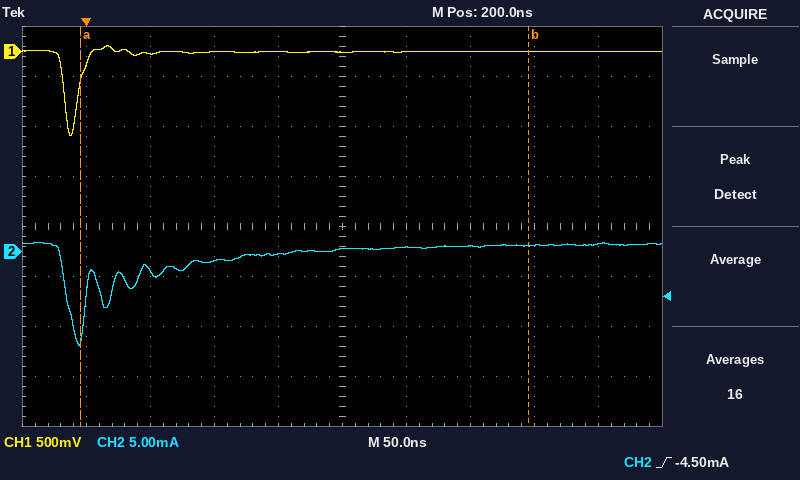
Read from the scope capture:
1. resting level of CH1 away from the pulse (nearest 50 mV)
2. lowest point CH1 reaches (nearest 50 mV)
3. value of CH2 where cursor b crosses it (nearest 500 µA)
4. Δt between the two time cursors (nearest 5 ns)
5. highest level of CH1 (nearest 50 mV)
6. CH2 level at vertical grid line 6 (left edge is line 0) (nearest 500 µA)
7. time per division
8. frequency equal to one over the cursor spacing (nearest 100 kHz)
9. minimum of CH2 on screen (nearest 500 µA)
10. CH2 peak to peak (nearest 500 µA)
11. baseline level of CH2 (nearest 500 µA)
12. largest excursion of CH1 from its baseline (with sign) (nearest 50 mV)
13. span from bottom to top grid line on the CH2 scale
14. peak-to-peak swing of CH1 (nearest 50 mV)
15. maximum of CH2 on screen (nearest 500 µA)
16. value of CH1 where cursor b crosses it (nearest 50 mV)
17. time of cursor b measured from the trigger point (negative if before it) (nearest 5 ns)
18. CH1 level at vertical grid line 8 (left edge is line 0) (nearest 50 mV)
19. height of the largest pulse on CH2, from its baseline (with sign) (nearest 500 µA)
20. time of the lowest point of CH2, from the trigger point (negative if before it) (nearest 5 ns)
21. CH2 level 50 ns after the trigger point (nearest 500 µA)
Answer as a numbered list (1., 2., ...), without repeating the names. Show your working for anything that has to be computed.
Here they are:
1. 0 mV
2. -850 mV
3. 500 µA
4. 350 ns
5. 50 mV
6. 500 µA
7. 50 ns
8. 1 / 350 ns ≈ 2.9 MHz
9. -9.5 mA
10. 1.0 mA − (-9.5 mA) = 10.5 mA
11. 500 µA
12. -850 mV − (0 mV) = -850 mV
13. 40 mA
14. 50 mV − (-850 mV) = 900 mV
15. 1.0 mA
16. 0 mV
17. +345 ns
18. 0 mV
19. -9.5 mA − (500 µA) = -10.0 mA
20. -5 ns
21. -2.0 mA
